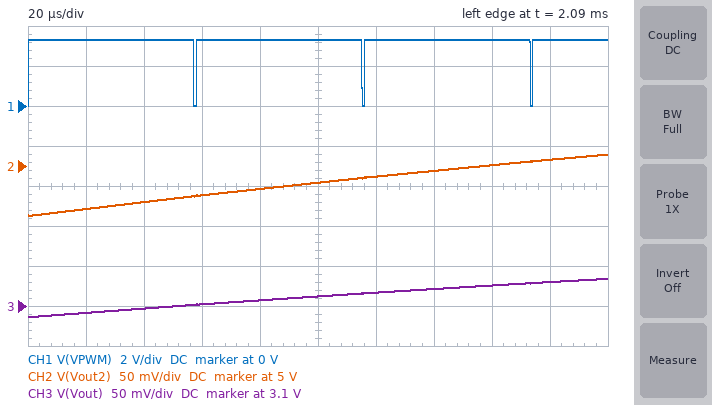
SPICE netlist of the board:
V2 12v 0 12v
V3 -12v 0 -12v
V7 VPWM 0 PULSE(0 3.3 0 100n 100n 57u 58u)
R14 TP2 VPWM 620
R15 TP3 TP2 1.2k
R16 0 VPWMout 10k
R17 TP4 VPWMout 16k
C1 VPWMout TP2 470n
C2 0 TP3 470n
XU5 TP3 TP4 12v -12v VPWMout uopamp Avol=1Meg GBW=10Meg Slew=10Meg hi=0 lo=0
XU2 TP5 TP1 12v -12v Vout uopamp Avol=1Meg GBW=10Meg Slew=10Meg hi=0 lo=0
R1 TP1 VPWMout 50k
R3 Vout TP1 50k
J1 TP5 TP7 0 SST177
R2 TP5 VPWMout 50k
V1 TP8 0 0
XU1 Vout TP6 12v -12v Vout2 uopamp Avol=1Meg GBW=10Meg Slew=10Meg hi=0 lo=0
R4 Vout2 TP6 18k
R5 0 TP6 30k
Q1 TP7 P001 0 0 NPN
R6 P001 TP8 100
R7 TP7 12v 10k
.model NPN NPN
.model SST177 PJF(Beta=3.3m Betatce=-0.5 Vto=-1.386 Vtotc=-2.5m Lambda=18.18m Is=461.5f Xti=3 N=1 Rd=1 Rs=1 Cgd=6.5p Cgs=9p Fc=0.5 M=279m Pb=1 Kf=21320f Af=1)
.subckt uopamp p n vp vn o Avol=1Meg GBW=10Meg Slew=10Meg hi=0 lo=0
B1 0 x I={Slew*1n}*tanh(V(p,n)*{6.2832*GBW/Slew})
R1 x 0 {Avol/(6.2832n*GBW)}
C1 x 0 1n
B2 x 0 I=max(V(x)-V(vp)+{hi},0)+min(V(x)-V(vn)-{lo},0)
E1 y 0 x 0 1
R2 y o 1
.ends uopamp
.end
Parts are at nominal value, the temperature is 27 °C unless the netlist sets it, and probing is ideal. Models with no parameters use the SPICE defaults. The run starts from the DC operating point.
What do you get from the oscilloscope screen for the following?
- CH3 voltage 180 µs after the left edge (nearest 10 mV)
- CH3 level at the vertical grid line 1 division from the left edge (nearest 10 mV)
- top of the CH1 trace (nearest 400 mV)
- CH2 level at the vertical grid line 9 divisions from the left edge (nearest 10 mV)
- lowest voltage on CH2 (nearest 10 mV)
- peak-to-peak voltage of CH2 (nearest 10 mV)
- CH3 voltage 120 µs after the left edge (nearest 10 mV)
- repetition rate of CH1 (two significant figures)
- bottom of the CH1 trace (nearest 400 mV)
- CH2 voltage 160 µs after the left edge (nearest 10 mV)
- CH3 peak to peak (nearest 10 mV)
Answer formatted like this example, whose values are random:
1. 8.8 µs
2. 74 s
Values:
1. 3.13 V
2. 3.09 V
3. 3.2 V
4. 5.01 V
5. 4.94 V
6. 80 mV
7. 3.12 V
8. 17 kHz
9. 0 V
10. 5.00 V
11. 50 mV
